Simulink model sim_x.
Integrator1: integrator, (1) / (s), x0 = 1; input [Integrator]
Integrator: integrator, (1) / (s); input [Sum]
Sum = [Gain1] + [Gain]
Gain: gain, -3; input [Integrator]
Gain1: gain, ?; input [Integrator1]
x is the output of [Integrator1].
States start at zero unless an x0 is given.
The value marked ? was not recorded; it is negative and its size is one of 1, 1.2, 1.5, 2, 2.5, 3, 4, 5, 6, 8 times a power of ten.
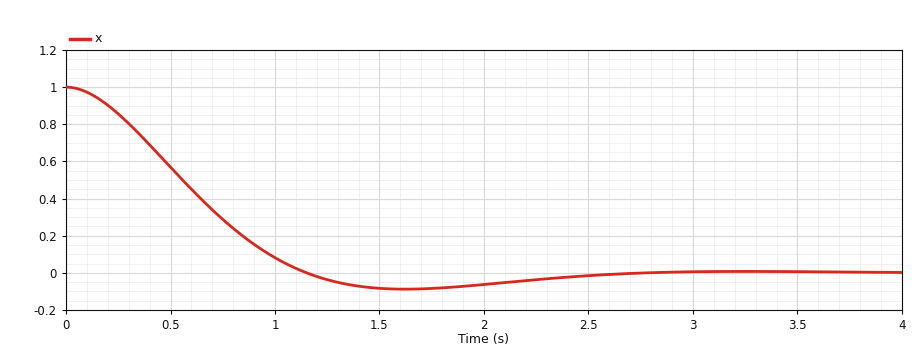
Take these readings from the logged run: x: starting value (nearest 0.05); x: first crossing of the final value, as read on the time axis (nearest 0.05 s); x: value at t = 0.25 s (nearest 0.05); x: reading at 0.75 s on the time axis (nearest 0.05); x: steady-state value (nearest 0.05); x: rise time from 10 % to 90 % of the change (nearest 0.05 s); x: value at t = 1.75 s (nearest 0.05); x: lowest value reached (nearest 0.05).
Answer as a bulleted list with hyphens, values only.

- 1.00
- 1.15 s
- 0.85
- 0.30
- 0.00
- 0.75 s
- -0.10
- -0.10
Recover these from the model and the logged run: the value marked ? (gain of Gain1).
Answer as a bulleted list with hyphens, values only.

- -6
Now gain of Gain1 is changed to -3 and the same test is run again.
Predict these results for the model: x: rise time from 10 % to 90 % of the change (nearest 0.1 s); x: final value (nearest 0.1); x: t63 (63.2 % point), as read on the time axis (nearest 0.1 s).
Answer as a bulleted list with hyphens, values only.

- 1.6 s
- 0.0
- 1.1 s
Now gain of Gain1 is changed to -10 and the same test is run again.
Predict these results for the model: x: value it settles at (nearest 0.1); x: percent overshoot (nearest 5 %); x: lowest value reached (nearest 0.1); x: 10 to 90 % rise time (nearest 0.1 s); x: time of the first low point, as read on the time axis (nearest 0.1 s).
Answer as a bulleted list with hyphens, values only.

- 0.0
- 20 %
- -0.2
- 0.5 s
- 1.1 s
